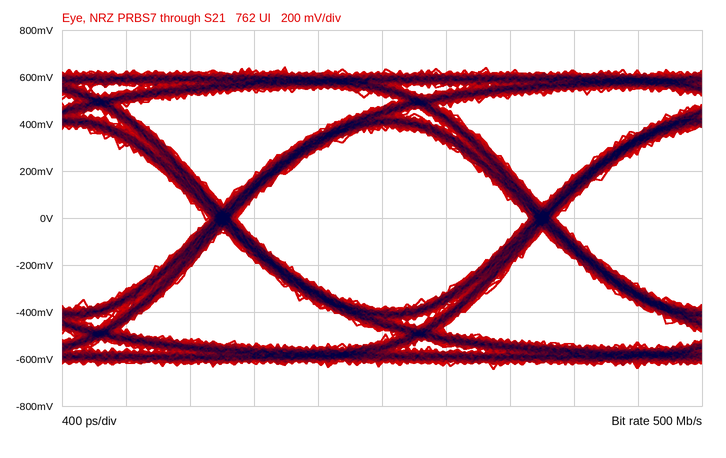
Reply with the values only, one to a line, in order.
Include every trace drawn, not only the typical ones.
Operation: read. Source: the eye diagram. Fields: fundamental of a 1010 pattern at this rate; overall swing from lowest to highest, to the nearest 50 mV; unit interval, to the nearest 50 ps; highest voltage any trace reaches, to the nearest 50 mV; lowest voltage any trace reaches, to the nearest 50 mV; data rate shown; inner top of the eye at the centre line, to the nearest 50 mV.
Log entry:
250 MHz
1.30 V
2.00 ns
650 mV
-650 mV
500 Mb/s
400 mV
